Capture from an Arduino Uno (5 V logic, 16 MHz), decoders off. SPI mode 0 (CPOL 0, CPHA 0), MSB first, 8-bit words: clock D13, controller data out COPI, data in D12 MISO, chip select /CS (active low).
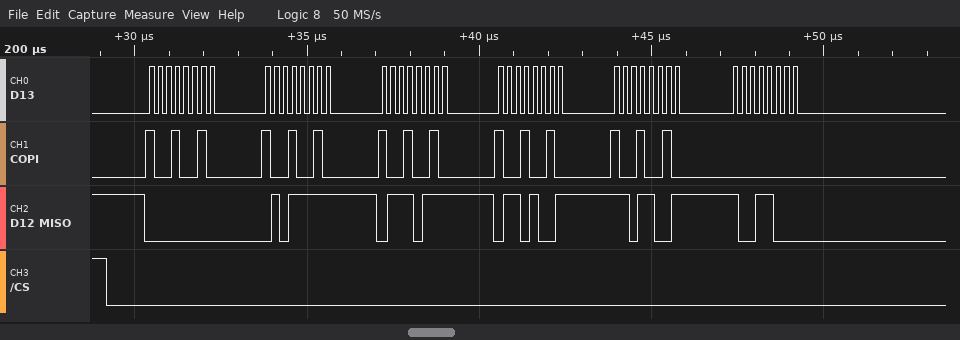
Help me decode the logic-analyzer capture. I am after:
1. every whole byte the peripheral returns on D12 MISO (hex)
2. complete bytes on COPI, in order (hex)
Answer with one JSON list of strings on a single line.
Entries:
["00 5F 77 69 D9 98", "92 92 92 92 92 00"]
